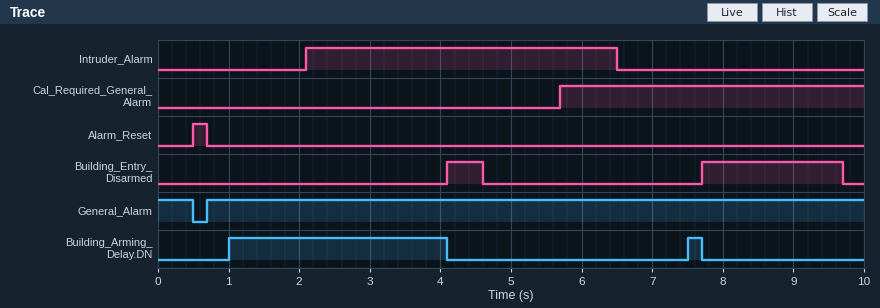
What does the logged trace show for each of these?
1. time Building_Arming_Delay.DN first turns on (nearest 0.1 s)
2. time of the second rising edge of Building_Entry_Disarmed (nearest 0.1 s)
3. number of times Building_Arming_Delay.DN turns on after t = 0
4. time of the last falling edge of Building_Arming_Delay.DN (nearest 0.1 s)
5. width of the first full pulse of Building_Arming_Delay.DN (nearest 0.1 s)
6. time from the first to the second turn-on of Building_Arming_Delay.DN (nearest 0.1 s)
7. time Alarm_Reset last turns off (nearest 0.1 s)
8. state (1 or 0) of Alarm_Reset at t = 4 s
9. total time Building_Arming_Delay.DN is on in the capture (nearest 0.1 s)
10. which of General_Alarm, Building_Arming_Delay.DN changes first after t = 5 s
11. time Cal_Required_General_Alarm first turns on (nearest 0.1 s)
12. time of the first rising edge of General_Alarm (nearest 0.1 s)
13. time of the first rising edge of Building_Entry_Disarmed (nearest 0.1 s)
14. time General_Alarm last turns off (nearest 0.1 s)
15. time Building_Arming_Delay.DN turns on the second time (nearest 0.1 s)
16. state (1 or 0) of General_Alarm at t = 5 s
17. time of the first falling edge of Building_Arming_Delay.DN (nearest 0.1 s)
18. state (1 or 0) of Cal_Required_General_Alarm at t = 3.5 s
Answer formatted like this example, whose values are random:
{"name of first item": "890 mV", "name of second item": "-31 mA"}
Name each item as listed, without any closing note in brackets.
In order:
{"time Building_Arming_Delay.DN first turns on": "1.0 s", "time of the second rising edge of Building_Entry_Disarmed": "7.7 s", "number of times Building_Arming_Delay.DN turns on after t = 0": "2", "time of the last falling edge of Building_Arming_Delay.DN": "7.7 s", "width of the first full pulse of Building_Arming_Delay.DN": "3.1 s", "time from the first to the second turn-on of Building_Arming_Delay.DN": "6.5 s", "time Alarm_Reset last turns off": "0.7 s", "state (1 or 0) of Alarm_Reset at t = 4 s": "0", "total time Building_Arming_Delay.DN is on in the capture": "3.3 s", "which of General_Alarm, Building_Arming_Delay.DN changes first after t = 5 s": "Building_Arming_Delay.DN", "time Cal_Required_General_Alarm first turns on": "5.7 s", "time of the first rising edge of General_Alarm": "0.7 s", "time of the first rising edge of Building_Entry_Disarmed": "4.1 s", "time General_Alarm last turns off": "0.5 s", "time Building_Arming_Delay.DN turns on the second time": "7.5 s", "state (1 or 0) of General_Alarm at t = 5 s": "1", "time of the first falling edge of Building_Arming_Delay.DN": "4.1 s", "state (1 or 0) of Cal_Required_General_Alarm at t = 3.5 s": "0"}
